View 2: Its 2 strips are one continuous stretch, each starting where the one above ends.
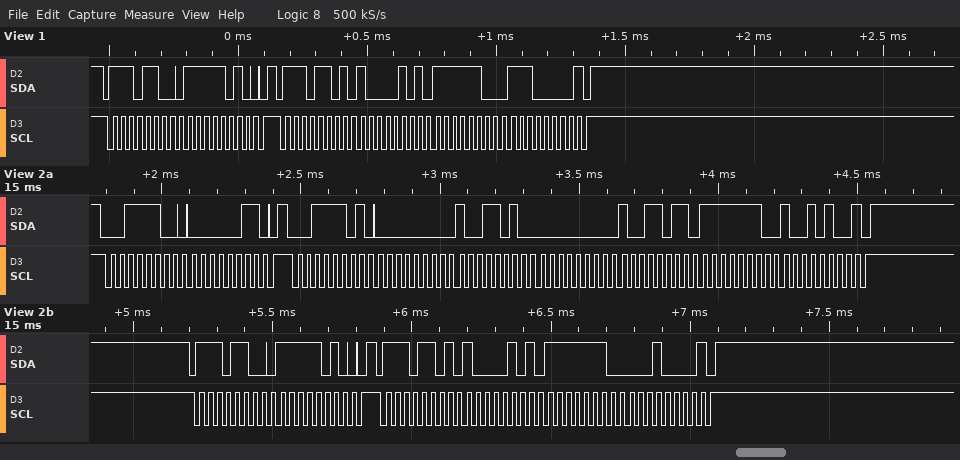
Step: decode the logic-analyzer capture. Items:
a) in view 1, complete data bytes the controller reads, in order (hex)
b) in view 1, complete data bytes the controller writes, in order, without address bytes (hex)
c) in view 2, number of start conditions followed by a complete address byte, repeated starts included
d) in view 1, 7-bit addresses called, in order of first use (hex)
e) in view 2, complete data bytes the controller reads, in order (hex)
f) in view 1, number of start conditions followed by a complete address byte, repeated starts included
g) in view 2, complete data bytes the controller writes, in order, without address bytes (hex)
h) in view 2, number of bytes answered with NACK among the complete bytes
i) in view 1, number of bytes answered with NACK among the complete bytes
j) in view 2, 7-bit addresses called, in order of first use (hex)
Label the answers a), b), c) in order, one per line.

a) 85 FC E0
b) FA
c) 4
d) 0x76
e) 00 9A 00 9B FE 94 85 FE 10
f) 2
g) 03 FA
h) 2
i) 1
j) 0x1E 0x76
